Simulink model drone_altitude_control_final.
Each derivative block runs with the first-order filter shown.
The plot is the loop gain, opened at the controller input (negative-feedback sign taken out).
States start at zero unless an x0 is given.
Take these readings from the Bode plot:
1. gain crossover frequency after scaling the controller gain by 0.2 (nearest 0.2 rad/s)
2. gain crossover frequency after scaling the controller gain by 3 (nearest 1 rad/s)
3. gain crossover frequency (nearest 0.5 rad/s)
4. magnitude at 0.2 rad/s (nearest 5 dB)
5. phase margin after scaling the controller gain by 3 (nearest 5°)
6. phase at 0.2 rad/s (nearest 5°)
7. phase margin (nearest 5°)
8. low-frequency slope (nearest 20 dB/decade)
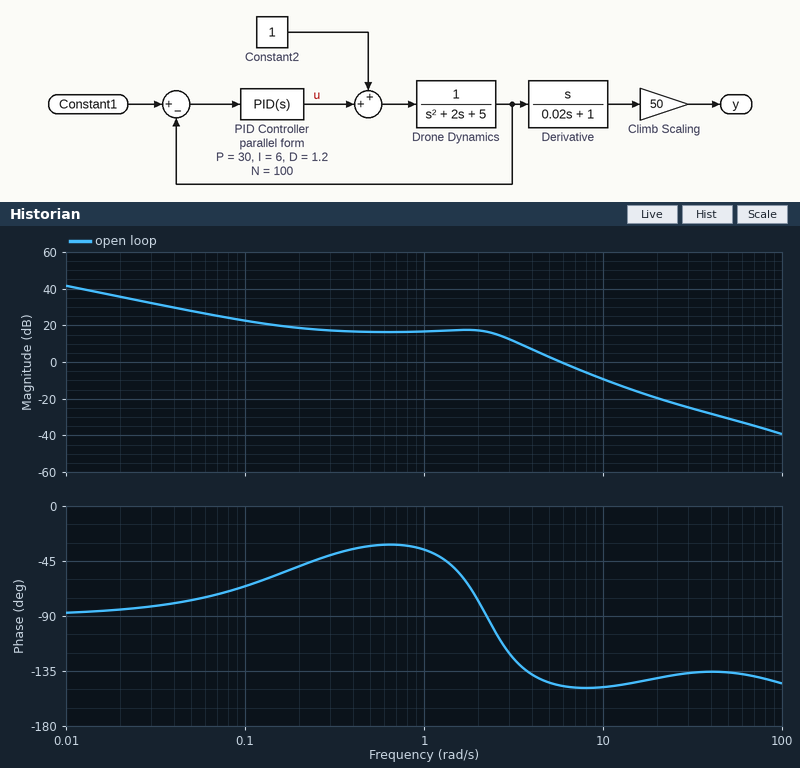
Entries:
2.8 rad/s
10 rad/s
6.0 rad/s
20 dB
30°
-50°
35°
-20 dB/decade
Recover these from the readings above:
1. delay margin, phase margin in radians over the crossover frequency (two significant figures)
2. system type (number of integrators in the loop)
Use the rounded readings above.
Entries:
0.10 s
1
